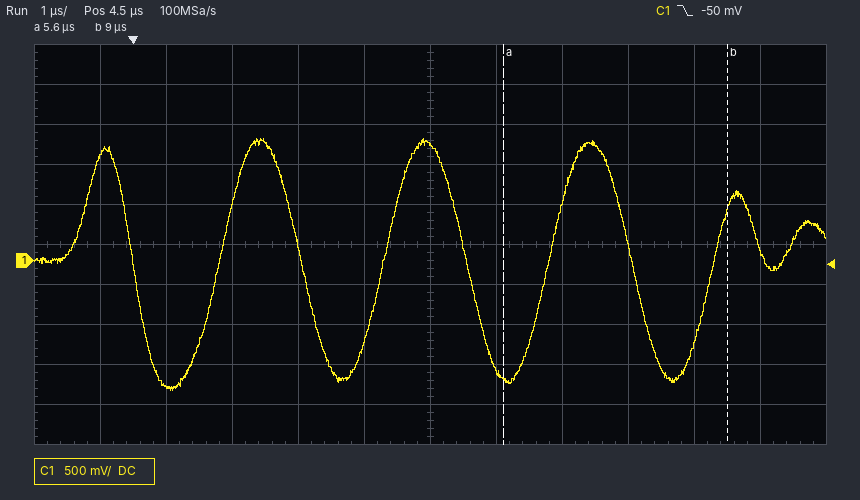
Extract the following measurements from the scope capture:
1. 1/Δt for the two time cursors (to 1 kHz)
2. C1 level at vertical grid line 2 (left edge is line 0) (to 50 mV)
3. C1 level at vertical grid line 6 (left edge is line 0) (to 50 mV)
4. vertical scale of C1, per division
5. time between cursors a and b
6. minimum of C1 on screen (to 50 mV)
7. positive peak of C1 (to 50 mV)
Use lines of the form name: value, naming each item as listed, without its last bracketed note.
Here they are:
1/Δt for the two time cursors: 294 kHz
C1 level at vertical grid line 2 (left edge is line 0): -1.55 V
C1 level at vertical grid line 6 (left edge is line 0): 1.45 V
vertical scale of C1, per division: 500 mV
time between cursors a and b: 3.4 µs
minimum of C1 on screen: -1.60 V
positive peak of C1: 1.50 V
